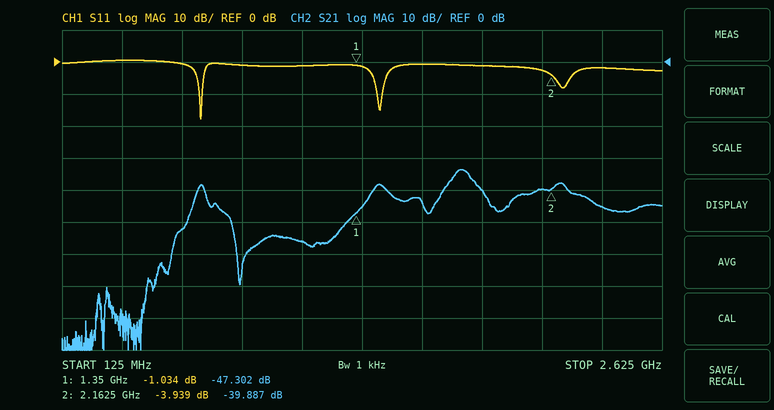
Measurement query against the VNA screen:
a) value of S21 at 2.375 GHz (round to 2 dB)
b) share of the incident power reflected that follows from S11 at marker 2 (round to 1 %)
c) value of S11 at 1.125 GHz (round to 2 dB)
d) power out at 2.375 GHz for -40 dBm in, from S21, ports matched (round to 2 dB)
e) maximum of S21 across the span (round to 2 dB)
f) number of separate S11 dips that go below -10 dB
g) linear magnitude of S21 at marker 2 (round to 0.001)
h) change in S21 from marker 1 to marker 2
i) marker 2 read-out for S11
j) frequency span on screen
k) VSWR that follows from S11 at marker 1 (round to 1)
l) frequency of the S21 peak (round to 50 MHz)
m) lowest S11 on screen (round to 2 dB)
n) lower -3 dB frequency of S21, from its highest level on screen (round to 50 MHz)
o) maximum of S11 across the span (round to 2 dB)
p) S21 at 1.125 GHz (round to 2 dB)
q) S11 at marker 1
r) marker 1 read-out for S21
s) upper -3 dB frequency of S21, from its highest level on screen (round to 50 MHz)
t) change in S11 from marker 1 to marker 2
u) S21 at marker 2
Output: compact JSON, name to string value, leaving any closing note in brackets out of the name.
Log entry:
{"value of S21 at 2.375 GHz": "-46 dB", "share of the incident power reflected that follows from S11 at marker 2": "40 %", "value of S11 at 1.125 GHz": "-2 dB", "power out at 2.375 GHz for -40 dBm in, from S21, ports matched": "-86 dBm", "maximum of S21 across the span": "-34 dB", "number of separate S11 dips that go below -10 dB": "2", "linear magnitude of S21 at marker 2": "0.010", "change in S21 from marker 1 to marker 2": "7.415 dB", "marker 2 read-out for S11": "-3.939 dB", "frequency span on screen": "2.5 GHz", "VSWR that follows from S11 at marker 1": "17", "frequency of the S21 peak": "1.80 GHz", "lowest S11 on screen": "-18 dB", "lower -3 dB frequency of S21, from its highest level on screen": "1.75 GHz", "maximum of S11 across the span": "0 dB", "S21 at 1.125 GHz": "-56 dB", "S11 at marker 1": "-1.034 dB", "marker 1 read-out for S21": "-47.302 dB", "upper -3 dB frequency of S21, from its highest level on screen": "1.85 GHz", "change in S11 from marker 1 to marker 2": "-2.905 dB", "S21 at marker 2": "-39.887 dB"}
